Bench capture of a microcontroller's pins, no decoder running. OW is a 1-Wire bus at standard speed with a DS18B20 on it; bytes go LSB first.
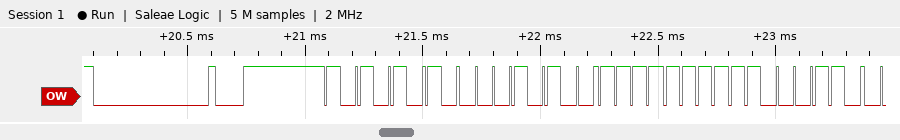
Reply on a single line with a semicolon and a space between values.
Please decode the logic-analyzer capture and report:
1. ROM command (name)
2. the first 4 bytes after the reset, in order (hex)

Match ROM; 55 28 FF 63
